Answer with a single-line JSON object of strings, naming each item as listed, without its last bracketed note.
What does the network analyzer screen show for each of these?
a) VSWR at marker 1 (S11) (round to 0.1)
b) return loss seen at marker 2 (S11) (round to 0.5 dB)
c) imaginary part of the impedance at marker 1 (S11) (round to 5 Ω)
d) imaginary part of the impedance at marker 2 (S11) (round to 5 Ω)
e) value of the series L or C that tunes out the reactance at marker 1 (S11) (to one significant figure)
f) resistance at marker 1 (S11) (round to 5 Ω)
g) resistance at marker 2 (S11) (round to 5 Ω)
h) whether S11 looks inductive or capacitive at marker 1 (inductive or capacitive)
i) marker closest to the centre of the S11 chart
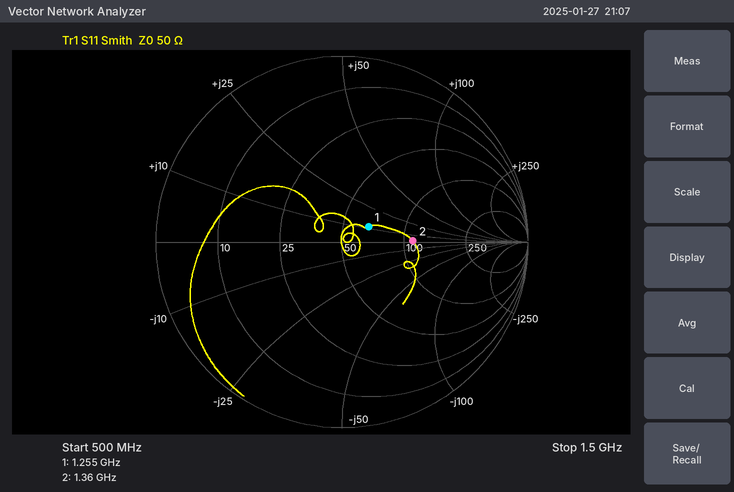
{"VSWR at marker 1 (S11)": "1.4", "return loss seen at marker 2 (S11)": "8.5 dB", "imaginary part of the impedance at marker 1 (S11)": "+10 Ω", "imaginary part of the impedance at marker 2 (S11)": "0 Ω", "value of the series L or C that tunes out the reactance at marker 1 (S11)": "10 pF", "resistance at marker 1 (S11)": "65 Ω", "resistance at marker 2 (S11)": "110 Ω", "whether S11 looks inductive or capacitive at marker 1": "inductive", "marker closest to the centre of the S11 chart": "marker 1"}
